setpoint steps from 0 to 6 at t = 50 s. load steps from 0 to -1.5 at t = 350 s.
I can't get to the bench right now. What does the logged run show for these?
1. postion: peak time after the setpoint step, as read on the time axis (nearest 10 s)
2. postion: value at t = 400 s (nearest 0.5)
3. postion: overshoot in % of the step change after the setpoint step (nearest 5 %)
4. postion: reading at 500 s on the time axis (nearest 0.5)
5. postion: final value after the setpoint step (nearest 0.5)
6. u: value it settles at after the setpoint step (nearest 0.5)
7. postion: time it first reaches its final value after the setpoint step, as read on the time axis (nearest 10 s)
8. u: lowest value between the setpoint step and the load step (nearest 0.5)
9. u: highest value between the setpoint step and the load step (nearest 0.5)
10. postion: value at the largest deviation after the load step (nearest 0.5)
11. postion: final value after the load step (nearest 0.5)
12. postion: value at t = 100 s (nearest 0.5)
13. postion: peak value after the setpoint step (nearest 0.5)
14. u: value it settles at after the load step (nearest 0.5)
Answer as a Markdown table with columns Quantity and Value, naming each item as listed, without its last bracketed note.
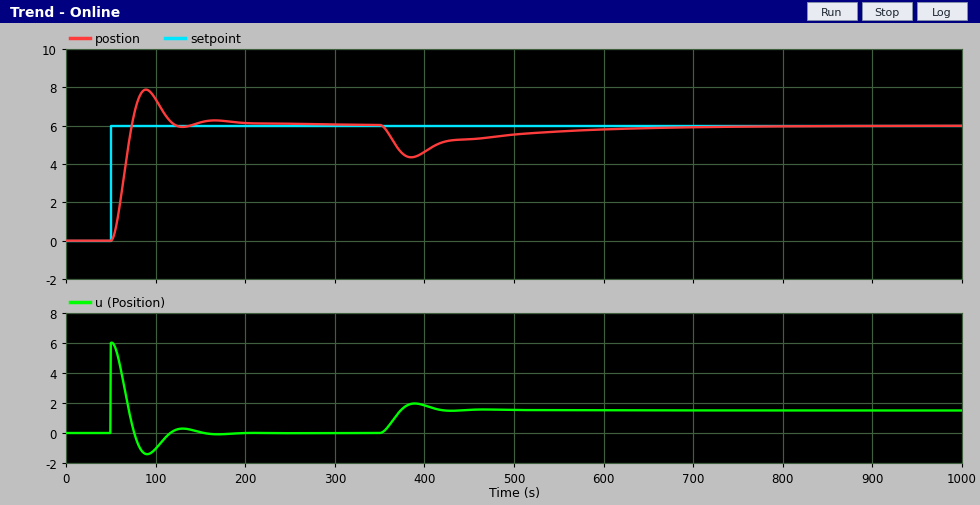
| Quantity | Value |
|---|---|
| postion: peak time after the setpoint step, as read on the time axis | 90 s |
| postion: value at t = 400 s | 4.5 |
| postion: overshoot in % of the step change after the setpoint step | 30 % |
| postion: reading at 500 s on the time axis | 5.5 |
| postion: final value after the setpoint step | 6.0 |
| u: value it settles at after the setpoint step | 0.0 |
| postion: time it first reaches its final value after the setpoint step, as read on the time axis | 70 s |
| u: lowest value between the setpoint step and the load step | -1.5 |
| u: highest value between the setpoint step and the load step | 6.0 |
| postion: value at the largest deviation after the load step | 4.5 |
| postion: final value after the load step | 6.0 |
| postion: value at t = 100 s | 7.5 |
| postion: peak value after the setpoint step | 8.0 |
| u: value it settles at after the load step | 1.5 |
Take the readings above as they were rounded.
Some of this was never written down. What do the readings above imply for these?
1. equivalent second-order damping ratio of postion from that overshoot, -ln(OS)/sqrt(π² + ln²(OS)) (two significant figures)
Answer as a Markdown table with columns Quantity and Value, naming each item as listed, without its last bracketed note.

| Quantity | Value |
|---|---|
| equivalent second-order damping ratio of postion from that overshoot, -ln(OS)/sqrt(π² + ln²(OS)) | 0.36 |
